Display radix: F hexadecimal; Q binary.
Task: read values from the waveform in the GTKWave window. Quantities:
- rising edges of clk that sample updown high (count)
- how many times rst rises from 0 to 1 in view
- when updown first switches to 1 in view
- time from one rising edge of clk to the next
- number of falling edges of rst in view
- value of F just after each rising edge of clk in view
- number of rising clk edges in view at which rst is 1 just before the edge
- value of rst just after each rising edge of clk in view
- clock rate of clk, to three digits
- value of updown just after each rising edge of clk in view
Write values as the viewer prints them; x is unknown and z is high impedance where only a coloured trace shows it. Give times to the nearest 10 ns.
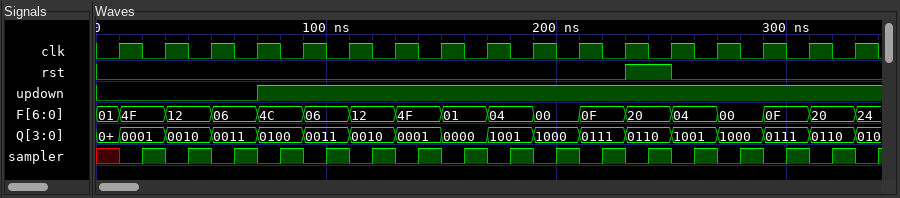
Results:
13
1
70 ns
20 ns
1
4F, 12, 06, 4C, 06, 12, 4F, 01, 04, 00, 0F, 20, 04, 00, 0F, 20, 24
1
0 0 0 0 0 0 0 0 0 0 0 1 0 0 0 0 0
50.0 MHz
0 0 0 1 1 1 1 1 1 1 1 1 1 1 1 1 1
